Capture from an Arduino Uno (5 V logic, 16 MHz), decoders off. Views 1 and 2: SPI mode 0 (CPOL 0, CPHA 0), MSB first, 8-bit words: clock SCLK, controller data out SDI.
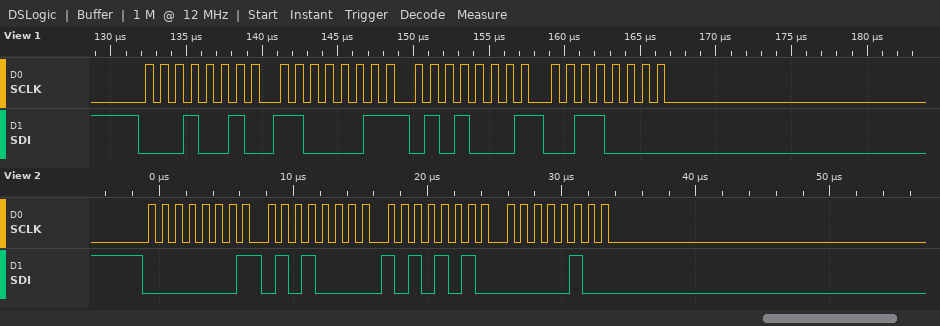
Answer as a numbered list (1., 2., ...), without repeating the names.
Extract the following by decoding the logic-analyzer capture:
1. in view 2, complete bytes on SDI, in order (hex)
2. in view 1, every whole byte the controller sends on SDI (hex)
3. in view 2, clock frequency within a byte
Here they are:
1. 01 50 AA 04
2. 12 C3 51 30
3. 1 MHz
